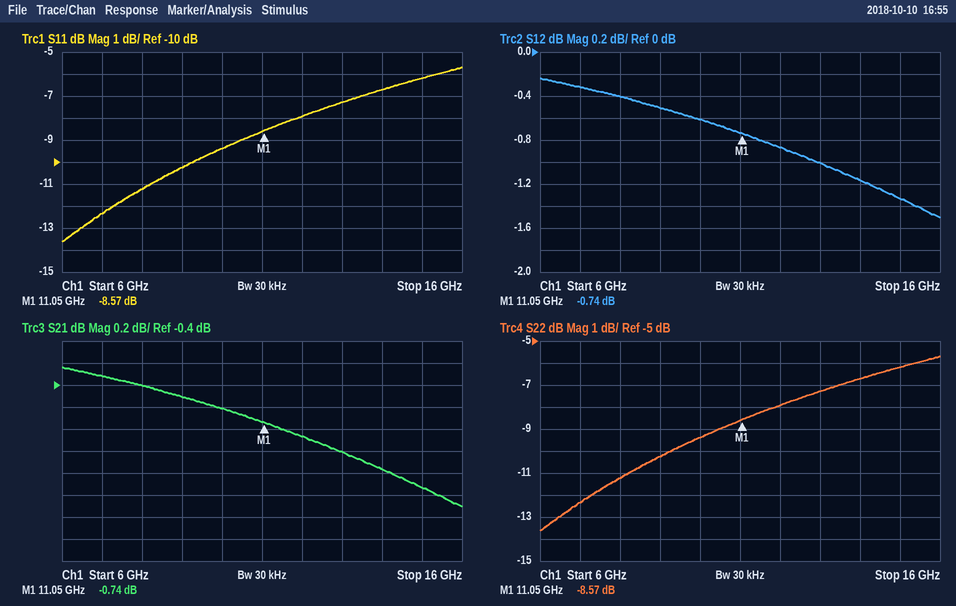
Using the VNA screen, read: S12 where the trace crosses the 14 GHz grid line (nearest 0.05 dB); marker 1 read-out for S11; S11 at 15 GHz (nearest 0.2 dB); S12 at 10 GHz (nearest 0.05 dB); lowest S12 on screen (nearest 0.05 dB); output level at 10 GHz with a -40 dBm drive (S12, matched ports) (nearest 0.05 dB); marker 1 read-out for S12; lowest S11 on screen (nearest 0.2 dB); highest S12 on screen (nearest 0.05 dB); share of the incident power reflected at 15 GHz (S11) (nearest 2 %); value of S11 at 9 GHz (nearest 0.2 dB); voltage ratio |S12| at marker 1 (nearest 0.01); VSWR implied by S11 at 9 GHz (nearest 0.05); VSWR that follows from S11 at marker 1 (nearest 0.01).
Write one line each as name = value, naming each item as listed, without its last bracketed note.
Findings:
S12 where the trace crosses the 14 GHz grid line = -1.15 dB
marker 1 read-out for S11 = -8.57 dB
S11 at 15 GHz = -6.2 dB
S12 at 10 GHz = -0.60 dB
lowest S12 on screen = -1.50 dB
output level at 10 GHz with a -40 dBm drive (S12, matched ports) = -40.60 dBm
marker 1 read-out for S12 = -0.74 dB
lowest S11 on screen = -13.6 dB
highest S12 on screen = -0.25 dB
share of the incident power reflected at 15 GHz (S11) = 24 %
value of S11 at 9 GHz = -10.2 dB
voltage ratio |S12| at marker 1 = 0.92
VSWR implied by S11 at 9 GHz = 1.90
VSWR that follows from S11 at marker 1 = 2.19
